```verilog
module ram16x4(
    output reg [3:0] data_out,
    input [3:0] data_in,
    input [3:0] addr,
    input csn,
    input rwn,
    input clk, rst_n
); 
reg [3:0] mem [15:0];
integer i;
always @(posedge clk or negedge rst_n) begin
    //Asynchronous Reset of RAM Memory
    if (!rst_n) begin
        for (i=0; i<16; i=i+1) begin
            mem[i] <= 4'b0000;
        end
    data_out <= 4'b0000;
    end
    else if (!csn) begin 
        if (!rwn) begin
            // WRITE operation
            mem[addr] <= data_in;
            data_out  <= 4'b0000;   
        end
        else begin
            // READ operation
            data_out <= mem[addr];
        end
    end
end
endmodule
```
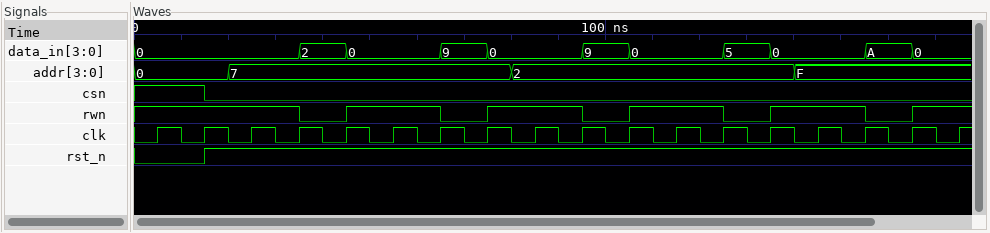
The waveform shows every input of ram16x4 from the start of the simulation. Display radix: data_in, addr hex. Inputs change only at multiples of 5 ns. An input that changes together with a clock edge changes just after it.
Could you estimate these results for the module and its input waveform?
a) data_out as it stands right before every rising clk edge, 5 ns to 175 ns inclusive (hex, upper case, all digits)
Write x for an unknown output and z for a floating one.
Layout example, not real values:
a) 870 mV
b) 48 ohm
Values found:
a) 0, 0, 0, 0, 0, 0, 2, 2, 0, 0, 0, 0, 9, 9, 0, 0, 0, 0
